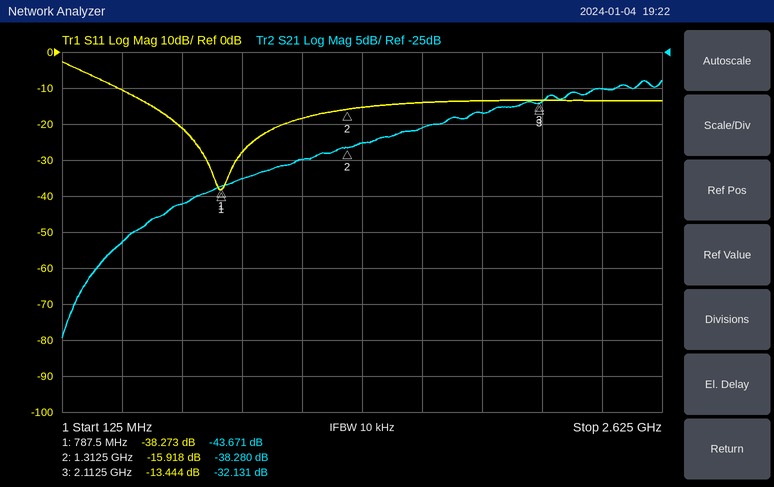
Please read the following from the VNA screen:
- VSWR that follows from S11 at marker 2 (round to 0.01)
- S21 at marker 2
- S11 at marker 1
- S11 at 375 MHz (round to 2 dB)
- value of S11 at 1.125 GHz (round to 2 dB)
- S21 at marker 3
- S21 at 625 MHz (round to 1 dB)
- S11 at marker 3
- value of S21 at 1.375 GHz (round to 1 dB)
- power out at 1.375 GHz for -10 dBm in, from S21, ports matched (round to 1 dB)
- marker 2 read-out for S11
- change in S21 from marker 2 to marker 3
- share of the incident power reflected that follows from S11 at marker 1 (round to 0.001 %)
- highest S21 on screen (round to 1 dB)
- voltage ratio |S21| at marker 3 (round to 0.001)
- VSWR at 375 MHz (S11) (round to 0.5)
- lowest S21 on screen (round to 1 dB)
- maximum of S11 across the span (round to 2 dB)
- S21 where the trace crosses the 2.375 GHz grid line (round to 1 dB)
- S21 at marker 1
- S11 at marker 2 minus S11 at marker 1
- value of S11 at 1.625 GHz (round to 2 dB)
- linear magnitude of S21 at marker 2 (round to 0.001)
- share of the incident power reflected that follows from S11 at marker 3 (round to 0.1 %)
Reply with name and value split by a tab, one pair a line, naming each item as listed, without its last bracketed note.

VSWR that follows from S11 at marker 2	1.38
S21 at marker 2	-38.280 dB
S11 at marker 1	-38.273 dB
S11 at 375 MHz	-10 dB
value of S11 at 1.125 GHz	-18 dB
S21 at marker 3	-32.131 dB
S21 at 625 MHz	-46 dB
S11 at marker 3	-13.444 dB
value of S21 at 1.375 GHz	-38 dB
power out at 1.375 GHz for -10 dBm in, from S21, ports matched	-48 dBm
marker 2 read-out for S11	-15.918 dB
change in S21 from marker 2 to marker 3	6.149 dB
share of the incident power reflected that follows from S11 at marker 1	0.015 %
highest S21 on screen	-29 dB
voltage ratio |S21| at marker 3	0.025
VSWR at 375 MHz (S11)	2.0
lowest S21 on screen	-65 dB
maximum of S11 across the span	-2 dB
S21 where the trace crosses the 2.375 GHz grid line	-30 dB
S21 at marker 1	-43.671 dB
S11 at marker 2 minus S11 at marker 1	22.355 dB
value of S11 at 1.625 GHz	-14 dB
linear magnitude of S21 at marker 2	0.012
share of the incident power reflected that follows from S11 at marker 3	4.5 %
